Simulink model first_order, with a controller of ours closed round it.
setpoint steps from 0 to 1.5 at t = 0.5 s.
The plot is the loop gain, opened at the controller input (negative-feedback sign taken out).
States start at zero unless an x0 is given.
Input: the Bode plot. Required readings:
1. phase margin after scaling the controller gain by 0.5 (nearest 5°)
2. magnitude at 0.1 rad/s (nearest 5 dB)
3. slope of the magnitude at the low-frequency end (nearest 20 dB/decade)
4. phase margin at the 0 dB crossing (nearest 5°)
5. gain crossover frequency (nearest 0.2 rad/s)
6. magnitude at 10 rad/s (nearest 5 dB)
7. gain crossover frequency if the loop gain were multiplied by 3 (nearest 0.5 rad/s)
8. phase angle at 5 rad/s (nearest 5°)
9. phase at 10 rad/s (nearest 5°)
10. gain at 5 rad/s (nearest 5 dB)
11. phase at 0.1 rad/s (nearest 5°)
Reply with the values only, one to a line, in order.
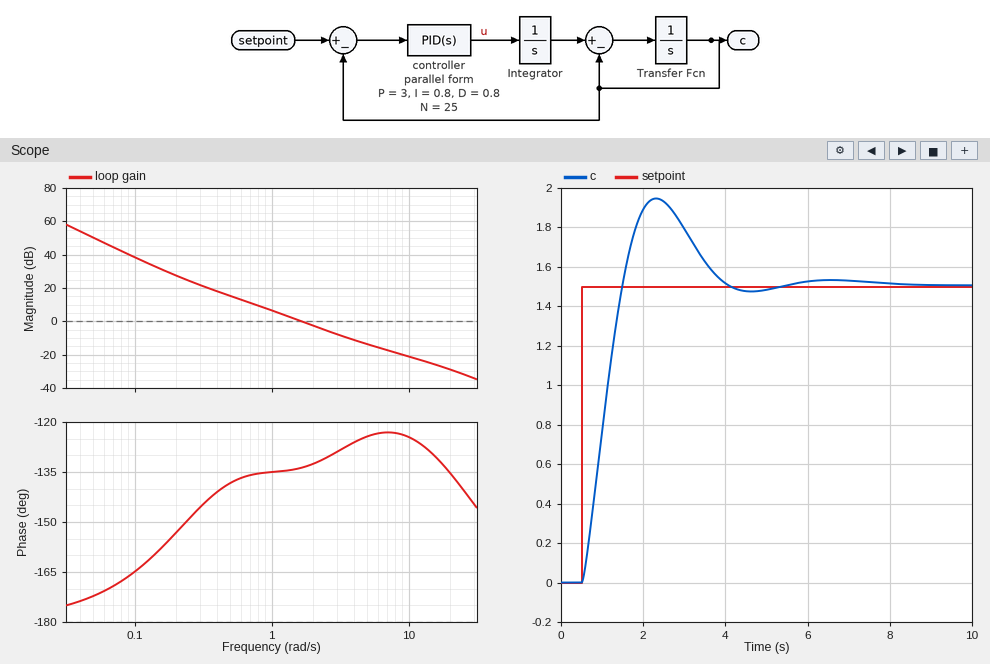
45°
40 dB
-40 dB/decade
45°
1.6 rad/s
-20 dB
3.5 rad/s
-125°
-125°
-15 dB
-165°
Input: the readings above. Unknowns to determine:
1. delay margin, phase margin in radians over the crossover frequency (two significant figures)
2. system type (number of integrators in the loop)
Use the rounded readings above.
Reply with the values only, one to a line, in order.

0.49 s
2
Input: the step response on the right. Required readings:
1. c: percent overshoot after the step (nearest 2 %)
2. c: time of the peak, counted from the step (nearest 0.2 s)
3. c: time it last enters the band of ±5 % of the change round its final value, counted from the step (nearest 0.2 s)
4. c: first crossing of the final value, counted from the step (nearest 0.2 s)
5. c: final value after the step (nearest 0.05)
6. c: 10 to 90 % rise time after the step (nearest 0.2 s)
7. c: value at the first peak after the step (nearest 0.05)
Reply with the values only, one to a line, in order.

30 %
1.8 s
3.2 s
1.0 s
1.50
0.8 s
1.95
